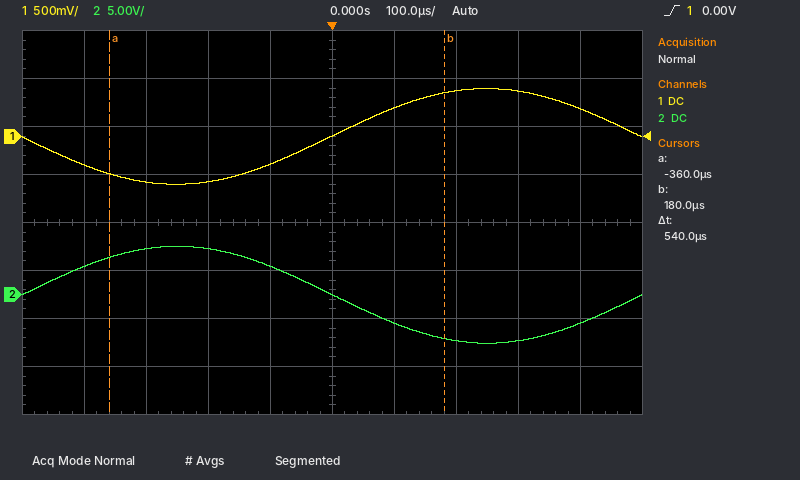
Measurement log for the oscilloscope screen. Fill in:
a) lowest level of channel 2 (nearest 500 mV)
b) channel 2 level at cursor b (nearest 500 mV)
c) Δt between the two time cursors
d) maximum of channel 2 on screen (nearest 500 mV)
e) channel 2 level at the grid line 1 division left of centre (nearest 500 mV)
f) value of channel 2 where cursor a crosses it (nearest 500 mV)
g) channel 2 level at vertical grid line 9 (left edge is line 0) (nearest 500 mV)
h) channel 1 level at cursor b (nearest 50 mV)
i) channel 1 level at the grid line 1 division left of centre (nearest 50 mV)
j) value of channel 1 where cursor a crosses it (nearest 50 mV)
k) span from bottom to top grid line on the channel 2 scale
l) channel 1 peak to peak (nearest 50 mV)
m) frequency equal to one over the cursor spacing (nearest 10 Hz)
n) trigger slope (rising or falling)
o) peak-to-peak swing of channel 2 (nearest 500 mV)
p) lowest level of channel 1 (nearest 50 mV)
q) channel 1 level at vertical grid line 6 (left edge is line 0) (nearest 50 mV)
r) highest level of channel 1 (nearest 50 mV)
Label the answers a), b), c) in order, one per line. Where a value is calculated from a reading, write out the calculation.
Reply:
a) -5.0 V
b) -4.5 V
c) 540 µs
d) 5.0 V
e) 3.0 V
f) 4.0 V
g) -3.0 V
h) 450 mV
i) -300 mV
j) -400 mV
k) 40 V
l) 500 mV − (-500 mV) = 1.00 V
m) 1 / 540 µs ≈ 1.85 kHz
n) rising
o) 5.0 V − (-5.0 V) = 10.0 V
p) -500 mV
q) 300 mV
r) 500 mV
